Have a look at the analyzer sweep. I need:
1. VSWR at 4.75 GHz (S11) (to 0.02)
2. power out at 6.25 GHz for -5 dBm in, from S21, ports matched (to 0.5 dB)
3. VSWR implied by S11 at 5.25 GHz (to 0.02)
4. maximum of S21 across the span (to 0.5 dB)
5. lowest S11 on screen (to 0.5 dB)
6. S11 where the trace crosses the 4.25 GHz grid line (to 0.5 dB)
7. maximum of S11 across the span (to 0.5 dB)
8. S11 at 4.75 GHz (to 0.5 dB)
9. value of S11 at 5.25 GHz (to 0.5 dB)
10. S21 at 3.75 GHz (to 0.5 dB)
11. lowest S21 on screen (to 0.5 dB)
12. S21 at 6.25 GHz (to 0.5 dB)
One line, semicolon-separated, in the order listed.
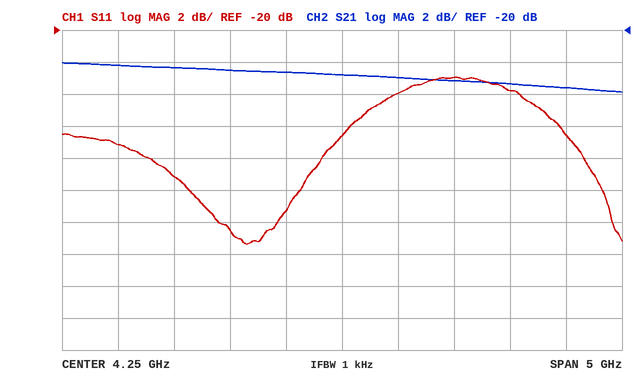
1.14; -28.5 dBm; 1.16; -22.0 dB; -33.5 dB; -26.5 dB; -23.0 dB; -24.0 dB; -23.0 dB; -22.5 dB; -24.0 dB; -23.5 dB
